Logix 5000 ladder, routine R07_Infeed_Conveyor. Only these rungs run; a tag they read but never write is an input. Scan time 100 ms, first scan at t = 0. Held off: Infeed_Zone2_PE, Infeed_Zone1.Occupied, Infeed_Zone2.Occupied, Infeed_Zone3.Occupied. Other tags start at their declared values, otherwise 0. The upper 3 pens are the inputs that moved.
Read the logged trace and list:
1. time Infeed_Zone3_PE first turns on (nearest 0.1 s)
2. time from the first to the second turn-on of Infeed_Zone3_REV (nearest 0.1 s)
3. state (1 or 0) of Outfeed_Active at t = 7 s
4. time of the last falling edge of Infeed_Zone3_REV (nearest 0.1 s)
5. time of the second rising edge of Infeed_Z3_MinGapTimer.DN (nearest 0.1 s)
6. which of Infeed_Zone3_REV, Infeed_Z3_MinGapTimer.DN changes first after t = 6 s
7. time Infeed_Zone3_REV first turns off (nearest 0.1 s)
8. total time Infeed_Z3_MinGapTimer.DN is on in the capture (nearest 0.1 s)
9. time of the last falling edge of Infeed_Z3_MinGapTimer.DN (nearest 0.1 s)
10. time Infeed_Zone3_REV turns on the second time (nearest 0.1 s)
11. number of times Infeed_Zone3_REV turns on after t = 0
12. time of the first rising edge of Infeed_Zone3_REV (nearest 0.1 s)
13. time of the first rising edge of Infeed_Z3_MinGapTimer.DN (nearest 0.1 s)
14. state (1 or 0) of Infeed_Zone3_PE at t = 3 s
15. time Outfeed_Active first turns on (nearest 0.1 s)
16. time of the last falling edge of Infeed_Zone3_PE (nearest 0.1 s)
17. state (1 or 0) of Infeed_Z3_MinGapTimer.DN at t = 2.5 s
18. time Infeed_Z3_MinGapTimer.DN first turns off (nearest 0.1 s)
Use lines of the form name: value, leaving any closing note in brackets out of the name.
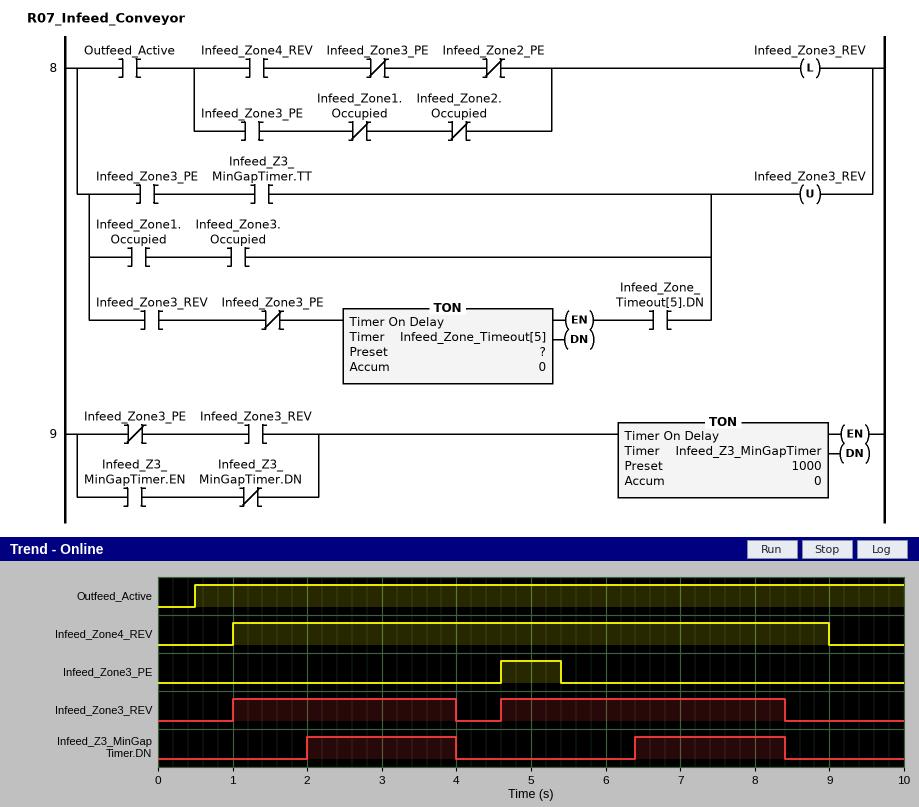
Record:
time Infeed_Zone3_PE first turns on: 4.6 s
time from the first to the second turn-on of Infeed_Zone3_REV: 3.6 s
state (1 or 0) of Outfeed_Active at t = 7 s: 1
time of the last falling edge of Infeed_Zone3_REV: 8.4 s
time of the second rising edge of Infeed_Z3_MinGapTimer.DN: 6.4 s
which of Infeed_Zone3_REV, Infeed_Z3_MinGapTimer.DN changes first after t = 6 s: Infeed_Z3_MinGapTimer.DN
time Infeed_Zone3_REV first turns off: 4.0 s
total time Infeed_Z3_MinGapTimer.DN is on in the capture: 4.0 s
time of the last falling edge of Infeed_Z3_MinGapTimer.DN: 8.4 s
time Infeed_Zone3_REV turns on the second time: 4.6 s
number of times Infeed_Zone3_REV turns on after t = 0: 2
time of the first rising edge of Infeed_Zone3_REV: 1.0 s
time of the first rising edge of Infeed_Z3_MinGapTimer.DN: 2.0 s
state (1 or 0) of Infeed_Zone3_PE at t = 3 s: 0
time Outfeed_Active first turns on: 0.5 s
time of the last falling edge of Infeed_Zone3_PE: 5.4 s
state (1 or 0) of Infeed_Z3_MinGapTimer.DN at t = 2.5 s: 1
time Infeed_Z3_MinGapTimer.DN first turns off: 4.0 s
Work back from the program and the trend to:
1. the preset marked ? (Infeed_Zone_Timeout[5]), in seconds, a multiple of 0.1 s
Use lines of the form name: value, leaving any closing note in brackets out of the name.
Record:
the preset marked ? (Infeed_Zone_Timeout[5]), in seconds, a multiple of 0.1 s: 3.0 s
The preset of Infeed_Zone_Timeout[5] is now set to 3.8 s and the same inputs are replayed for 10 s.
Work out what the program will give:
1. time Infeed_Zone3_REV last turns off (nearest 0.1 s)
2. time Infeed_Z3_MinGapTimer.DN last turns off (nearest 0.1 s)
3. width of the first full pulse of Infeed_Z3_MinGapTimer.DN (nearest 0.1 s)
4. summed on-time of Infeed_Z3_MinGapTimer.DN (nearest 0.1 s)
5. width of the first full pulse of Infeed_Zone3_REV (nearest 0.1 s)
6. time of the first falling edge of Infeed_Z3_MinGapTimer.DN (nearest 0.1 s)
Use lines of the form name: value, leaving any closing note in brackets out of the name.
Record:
time Infeed_Zone3_REV last turns off: 9.2 s
time Infeed_Z3_MinGapTimer.DN last turns off: 9.2 s
width of the first full pulse of Infeed_Z3_MinGapTimer.DN: 2.6 s
summed on-time of Infeed_Z3_MinGapTimer.DN: 5.4 s
width of the first full pulse of Infeed_Zone3_REV: 8.2 s
time of the first falling edge of Infeed_Z3_MinGapTimer.DN: 4.6 s
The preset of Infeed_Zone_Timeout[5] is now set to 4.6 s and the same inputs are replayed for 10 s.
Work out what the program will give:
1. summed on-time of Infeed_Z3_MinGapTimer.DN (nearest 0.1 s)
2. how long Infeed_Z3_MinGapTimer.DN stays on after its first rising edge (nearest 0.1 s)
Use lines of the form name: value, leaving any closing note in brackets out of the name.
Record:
summed on-time of Infeed_Z3_MinGapTimer.DN: 6.2 s
how long Infeed_Z3_MinGapTimer.DN stays on after its first rising edge: 2.6 s
